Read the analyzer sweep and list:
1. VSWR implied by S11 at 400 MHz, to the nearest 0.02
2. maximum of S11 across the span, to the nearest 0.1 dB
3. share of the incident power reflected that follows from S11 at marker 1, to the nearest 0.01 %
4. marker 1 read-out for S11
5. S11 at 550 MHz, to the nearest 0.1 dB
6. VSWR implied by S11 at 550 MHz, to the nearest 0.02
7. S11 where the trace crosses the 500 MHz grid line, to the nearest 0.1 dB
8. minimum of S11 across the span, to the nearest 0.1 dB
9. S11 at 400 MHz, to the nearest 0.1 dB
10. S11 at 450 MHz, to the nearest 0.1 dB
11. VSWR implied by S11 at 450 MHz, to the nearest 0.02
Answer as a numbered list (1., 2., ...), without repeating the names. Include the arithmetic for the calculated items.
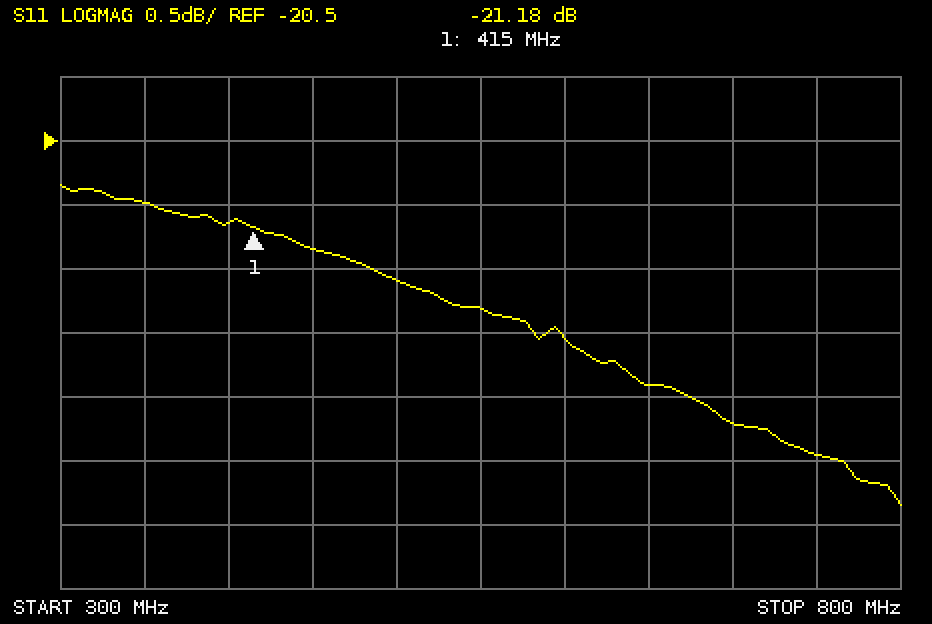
1. |Γ| = 10^(-21.1/20) = 0.0881; VSWR = (1 + 0.0881)/(1 − 0.0881) ≈ 1.19, so 1.20 to the nearest 0.02
2. -20.8 dB
3. 10^(-21.18/10) ≈ 0.76 %
4. -21.18 dB
5. -21.8 dB
6. |Γ| = 10^(-21.8/20) = 0.0813; VSWR = (1 + 0.0813)/(1 − 0.0813) ≈ 1.18
7. -21.6 dB
8. -23.3 dB
9. -21.1 dB
10. -21.3 dB
11. |Γ| = 10^(-21.3/20) = 0.0861; VSWR = (1 + 0.0861)/(1 − 0.0861) ≈ 1.19, so 1.18 to the nearest 0.02
